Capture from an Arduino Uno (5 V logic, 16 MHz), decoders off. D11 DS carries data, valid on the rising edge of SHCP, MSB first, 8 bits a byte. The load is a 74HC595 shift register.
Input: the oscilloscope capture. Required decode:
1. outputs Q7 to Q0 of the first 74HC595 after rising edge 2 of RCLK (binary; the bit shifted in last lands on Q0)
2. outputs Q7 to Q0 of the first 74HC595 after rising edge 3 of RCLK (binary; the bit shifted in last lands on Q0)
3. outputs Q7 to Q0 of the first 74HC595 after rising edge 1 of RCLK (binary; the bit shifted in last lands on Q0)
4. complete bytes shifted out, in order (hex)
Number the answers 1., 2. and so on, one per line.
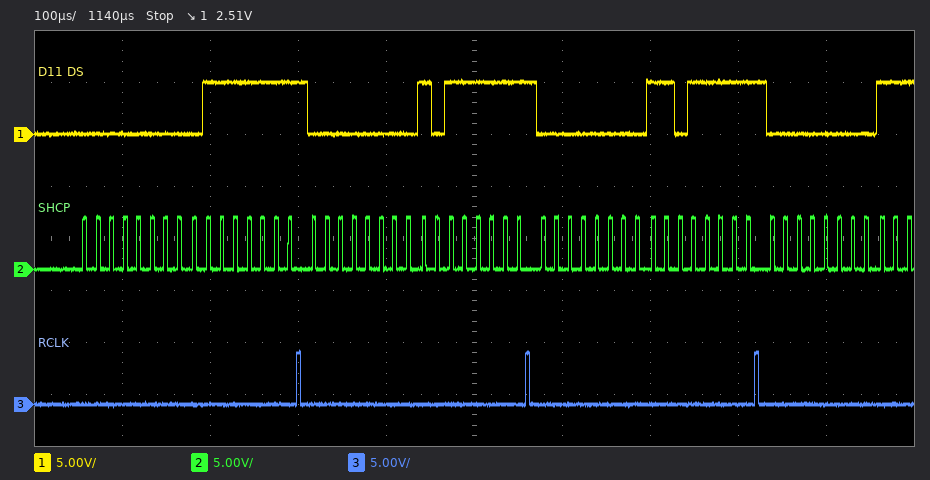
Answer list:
1. 10111111
2. 11011111
3. 01111111
4. 0x00 0x7F 0x00 0xBF 0x00 0xDF 0x00
